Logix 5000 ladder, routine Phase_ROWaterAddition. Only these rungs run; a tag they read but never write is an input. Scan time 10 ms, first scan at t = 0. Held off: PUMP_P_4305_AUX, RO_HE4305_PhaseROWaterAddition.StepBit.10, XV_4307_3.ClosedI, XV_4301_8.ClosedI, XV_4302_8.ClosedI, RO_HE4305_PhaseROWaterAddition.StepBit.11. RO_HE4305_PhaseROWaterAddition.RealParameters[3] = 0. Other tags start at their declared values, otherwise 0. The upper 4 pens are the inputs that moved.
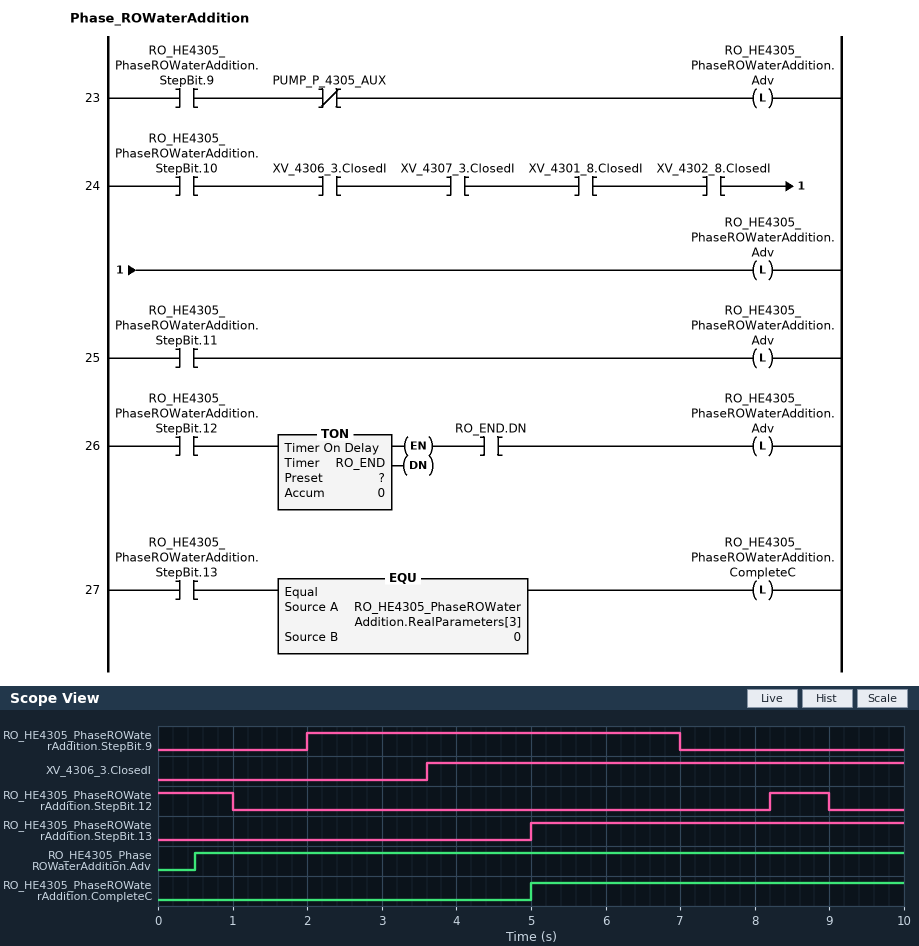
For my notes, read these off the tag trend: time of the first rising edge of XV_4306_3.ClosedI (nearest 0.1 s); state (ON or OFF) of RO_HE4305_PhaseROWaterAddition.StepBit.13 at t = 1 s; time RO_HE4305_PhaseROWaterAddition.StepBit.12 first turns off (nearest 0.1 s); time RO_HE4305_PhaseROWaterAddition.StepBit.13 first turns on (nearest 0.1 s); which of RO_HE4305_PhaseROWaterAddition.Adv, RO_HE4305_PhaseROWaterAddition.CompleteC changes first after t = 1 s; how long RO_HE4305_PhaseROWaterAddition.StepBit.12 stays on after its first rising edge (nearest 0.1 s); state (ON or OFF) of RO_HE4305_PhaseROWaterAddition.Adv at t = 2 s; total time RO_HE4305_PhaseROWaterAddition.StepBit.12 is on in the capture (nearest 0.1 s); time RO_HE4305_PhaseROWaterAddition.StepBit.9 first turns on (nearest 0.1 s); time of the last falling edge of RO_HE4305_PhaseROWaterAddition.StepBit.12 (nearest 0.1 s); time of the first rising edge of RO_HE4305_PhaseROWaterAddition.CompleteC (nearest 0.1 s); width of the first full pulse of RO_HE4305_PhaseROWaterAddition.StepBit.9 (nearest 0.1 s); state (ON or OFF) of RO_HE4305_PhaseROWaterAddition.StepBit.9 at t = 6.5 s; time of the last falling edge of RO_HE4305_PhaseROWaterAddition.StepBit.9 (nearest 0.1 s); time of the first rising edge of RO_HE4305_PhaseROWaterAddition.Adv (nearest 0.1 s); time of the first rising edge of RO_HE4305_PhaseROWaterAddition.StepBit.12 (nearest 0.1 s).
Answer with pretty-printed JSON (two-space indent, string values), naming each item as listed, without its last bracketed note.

{
  "time of the first rising edge of XV_4306_3.ClosedI": "3.6 s",
  "state (ON or OFF) of RO_HE4305_PhaseROWaterAddition.StepBit.13 at t = 1 s": "OFF",
  "time RO_HE4305_PhaseROWaterAddition.StepBit.12 first turns off": "1.0 s",
  "time RO_HE4305_PhaseROWaterAddition.StepBit.13 first turns on": "5.0 s",
  "which of RO_HE4305_PhaseROWaterAddition.Adv, RO_HE4305_PhaseROWaterAddition.CompleteC changes first after t = 1 s": "RO_HE4305_PhaseROWaterAddition.CompleteC",
  "how long RO_HE4305_PhaseROWaterAddition.StepBit.12 stays on after its first rising edge": "0.8 s",
  "state (ON or OFF) of RO_HE4305_PhaseROWaterAddition.Adv at t = 2 s": "ON",
  "total time RO_HE4305_PhaseROWaterAddition.StepBit.12 is on in the capture": "1.8 s",
  "time RO_HE4305_PhaseROWaterAddition.StepBit.9 first turns on": "2.0 s",
  "time of the last falling edge of RO_HE4305_PhaseROWaterAddition.StepBit.12": "9.0 s",
  "time of the first rising edge of RO_HE4305_PhaseROWaterAddition.CompleteC": "5.0 s",
  "width of the first full pulse of RO_HE4305_PhaseROWaterAddition.StepBit.9": "5.0 s",
  "state (ON or OFF) of RO_HE4305_PhaseROWaterAddition.StepBit.9 at t = 6.5 s": "ON",
  "time of the last falling edge of RO_HE4305_PhaseROWaterAddition.StepBit.9": "7.0 s",
  "time of the first rising edge of RO_HE4305_PhaseROWaterAddition.Adv": "0.5 s",
  "time of the first rising edge of RO_HE4305_PhaseROWaterAddition.StepBit.12": "8.2 s"
}
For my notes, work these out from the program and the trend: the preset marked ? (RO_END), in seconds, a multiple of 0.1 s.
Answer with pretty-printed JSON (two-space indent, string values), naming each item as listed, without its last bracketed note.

{
  "the preset marked ? (RO_END), in seconds, a multiple of 0.1 s": "0.5 s"
}
